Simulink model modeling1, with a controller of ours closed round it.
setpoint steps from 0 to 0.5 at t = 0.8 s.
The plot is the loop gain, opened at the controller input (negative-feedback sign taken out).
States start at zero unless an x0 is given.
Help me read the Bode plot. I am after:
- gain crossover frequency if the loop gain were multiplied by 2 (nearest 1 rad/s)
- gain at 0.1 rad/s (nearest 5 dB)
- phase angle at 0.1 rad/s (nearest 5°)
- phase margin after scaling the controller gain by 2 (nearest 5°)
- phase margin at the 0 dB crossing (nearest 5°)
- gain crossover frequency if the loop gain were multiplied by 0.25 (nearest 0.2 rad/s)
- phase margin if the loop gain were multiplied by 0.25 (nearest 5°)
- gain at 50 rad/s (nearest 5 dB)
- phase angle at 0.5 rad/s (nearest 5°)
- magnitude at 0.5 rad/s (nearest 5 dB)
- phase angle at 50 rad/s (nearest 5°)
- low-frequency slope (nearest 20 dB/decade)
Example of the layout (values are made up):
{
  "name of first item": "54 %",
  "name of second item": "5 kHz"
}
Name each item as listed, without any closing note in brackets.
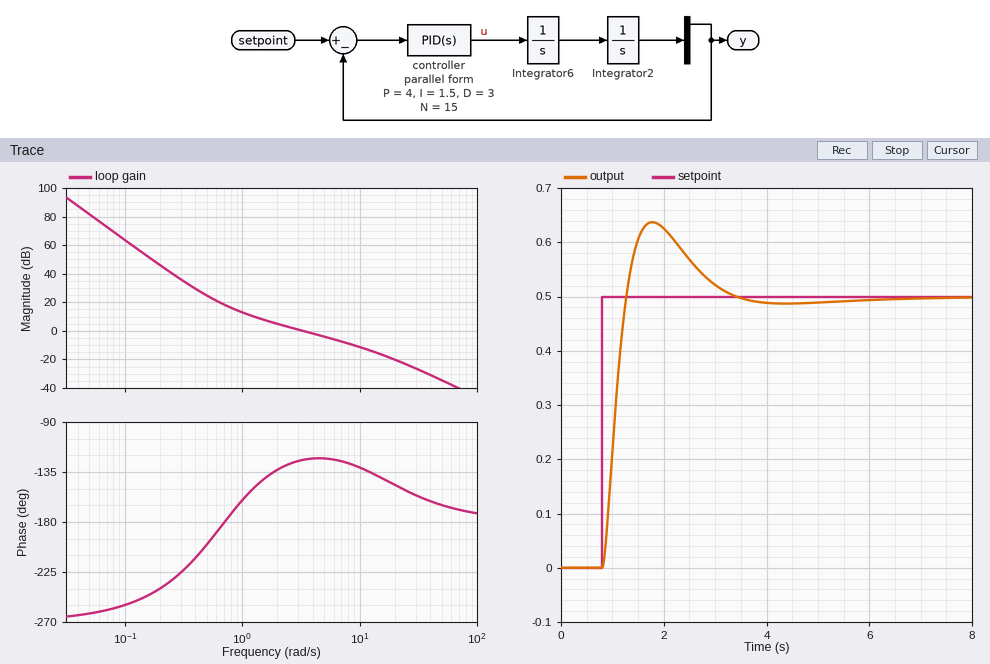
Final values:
{
  "gain crossover frequency if the loop gain were multiplied by 2": "6 rad/s",
  "gain at 0.1 rad/s": "65 dB",
  "phase angle at 0.1 rad/s": "-255°",
  "phase margin after scaling the controller gain by 2": "55°",
  "phase margin at the 0 dB crossing": "55°",
  "gain crossover frequency if the loop gain were multiplied by 0.25": "1.0 rad/s",
  "phase margin if the loop gain were multiplied by 0.25": "25°",
  "gain at 50 rad/s": "-35 dB",
  "phase angle at 0.5 rad/s": "-200°",
  "magnitude at 0.5 rad/s": "25 dB",
  "phase angle at 50 rad/s": "-165°",
  "low-frequency slope": "-60 dB/decade"
}
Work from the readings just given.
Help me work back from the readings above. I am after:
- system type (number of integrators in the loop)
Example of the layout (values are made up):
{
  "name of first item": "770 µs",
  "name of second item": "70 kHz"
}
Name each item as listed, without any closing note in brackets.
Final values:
{
  "system type": "3"
}
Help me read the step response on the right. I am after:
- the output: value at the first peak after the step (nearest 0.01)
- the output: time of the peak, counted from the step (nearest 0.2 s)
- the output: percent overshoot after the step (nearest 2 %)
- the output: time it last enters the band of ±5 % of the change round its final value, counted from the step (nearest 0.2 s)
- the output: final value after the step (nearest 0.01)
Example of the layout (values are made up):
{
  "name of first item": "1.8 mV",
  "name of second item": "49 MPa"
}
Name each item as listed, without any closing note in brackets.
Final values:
{
  "the output: value at the first peak after the step": "0.64",
  "the output: time of the peak, counted from the step": "1.0 s",
  "the output: percent overshoot after the step": "28 %",
  "the output: time it last enters the band of ±5 % of the change round its final value, counted from the step": "2.2 s",
  "the output: final value after the step": "0.50"
}
